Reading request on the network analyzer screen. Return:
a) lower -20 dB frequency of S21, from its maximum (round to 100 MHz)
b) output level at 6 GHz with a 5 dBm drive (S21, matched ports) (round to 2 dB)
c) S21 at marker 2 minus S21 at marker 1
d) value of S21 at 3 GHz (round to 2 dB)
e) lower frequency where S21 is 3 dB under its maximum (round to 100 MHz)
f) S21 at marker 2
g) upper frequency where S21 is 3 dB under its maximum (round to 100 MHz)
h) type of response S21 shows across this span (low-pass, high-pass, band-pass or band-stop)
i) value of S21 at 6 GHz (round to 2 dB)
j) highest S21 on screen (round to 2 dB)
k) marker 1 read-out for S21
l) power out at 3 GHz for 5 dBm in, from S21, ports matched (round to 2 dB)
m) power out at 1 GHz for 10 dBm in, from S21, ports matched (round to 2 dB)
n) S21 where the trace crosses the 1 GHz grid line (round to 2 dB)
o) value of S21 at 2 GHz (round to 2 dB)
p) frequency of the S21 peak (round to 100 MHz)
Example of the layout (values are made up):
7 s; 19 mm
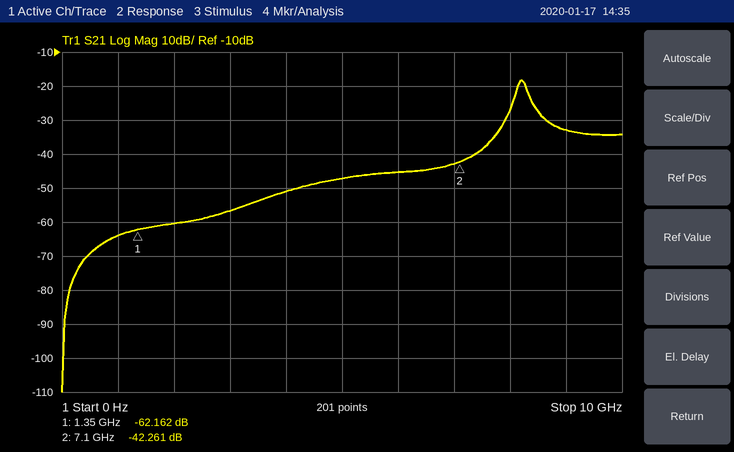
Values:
7.5 GHz; -40 dBm; 19.901 dB; -56 dB; 8.1 GHz; -42.261 dB; 8.3 GHz; band-pass; -46 dB; -18 dB; -62.162 dB; -52 dBm; -54 dBm; -64 dB; -60 dB; 8.2 GHz
